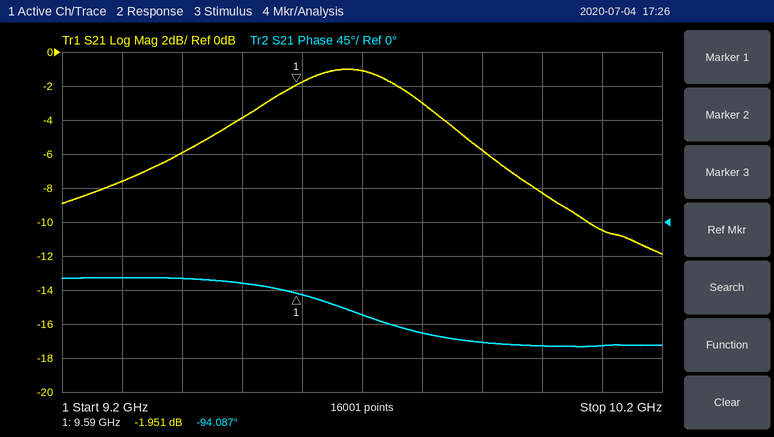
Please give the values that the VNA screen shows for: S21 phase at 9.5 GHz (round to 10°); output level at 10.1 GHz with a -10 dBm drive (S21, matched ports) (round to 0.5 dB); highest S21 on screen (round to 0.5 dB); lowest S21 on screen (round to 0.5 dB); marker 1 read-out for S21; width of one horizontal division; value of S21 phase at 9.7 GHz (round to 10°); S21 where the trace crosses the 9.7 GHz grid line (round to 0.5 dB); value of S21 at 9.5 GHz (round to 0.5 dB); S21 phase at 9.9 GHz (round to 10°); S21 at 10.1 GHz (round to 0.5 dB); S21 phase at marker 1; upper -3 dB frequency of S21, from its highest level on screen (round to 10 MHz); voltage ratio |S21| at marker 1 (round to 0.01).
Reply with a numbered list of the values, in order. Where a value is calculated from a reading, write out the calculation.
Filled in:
1. -80°
2. -10 dBm + (-10.5 dB) = -20.5 dBm
3. -1.0 dB
4. -12.0 dB
5. -1.951 dB
6. 100 MHz
7. -120°
8. -1.0 dB
9. -4.0 dB
10. -160°
11. -10.5 dB
12. -94.087°
13. 9.84 GHz
14. 10^(-1.951/20) ≈ 0.80
